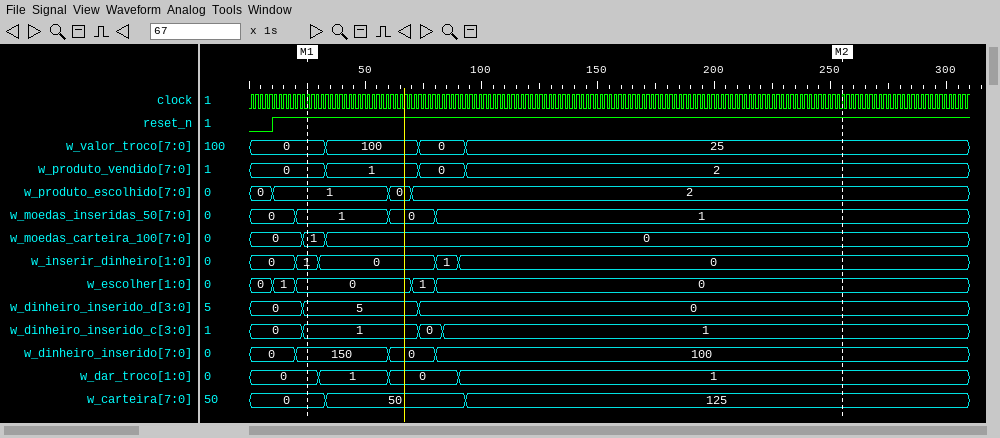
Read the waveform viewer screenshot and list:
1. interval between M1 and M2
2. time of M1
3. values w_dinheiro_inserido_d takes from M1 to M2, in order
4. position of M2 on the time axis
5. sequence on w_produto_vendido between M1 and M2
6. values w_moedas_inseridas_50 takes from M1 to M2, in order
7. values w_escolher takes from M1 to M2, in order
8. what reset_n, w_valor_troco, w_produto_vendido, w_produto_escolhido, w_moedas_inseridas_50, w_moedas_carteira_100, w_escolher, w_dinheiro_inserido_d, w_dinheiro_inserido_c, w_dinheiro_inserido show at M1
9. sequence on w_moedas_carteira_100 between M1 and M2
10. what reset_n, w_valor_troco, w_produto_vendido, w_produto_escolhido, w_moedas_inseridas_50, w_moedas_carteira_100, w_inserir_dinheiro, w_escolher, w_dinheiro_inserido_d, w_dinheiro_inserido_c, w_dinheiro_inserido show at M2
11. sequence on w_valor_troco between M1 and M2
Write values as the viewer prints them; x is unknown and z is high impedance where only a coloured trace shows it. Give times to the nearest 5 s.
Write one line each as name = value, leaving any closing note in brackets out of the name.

interval between M1 and M2 = 230 s
time of M1 = 25 s
values w_dinheiro_inserido_d takes from M1 to M2, in order = 5, 0
position of M2 on the time axis = 255 s
sequence on w_produto_vendido between M1 and M2 = 0, 1, 0, 2
values w_moedas_inseridas_50 takes from M1 to M2, in order = 1, 0, 1
values w_escolher takes from M1 to M2, in order = 0, 1, 0
what reset_n, w_valor_troco, w_produto_vendido, w_produto_escolhido, w_moedas_inseridas_50, w_moedas_carteira_100, w_escolher, w_dinheiro_inserido_d, w_dinheiro_inserido_c, w_dinheiro_inserido show at M1 = reset_n=1, w_valor_troco=0, w_produto_vendido=0, w_produto_escolhido=1, w_moedas_inseridas_50=1, w_moedas_carteira_100=1, w_escolher=0, w_dinheiro_inserido_d=5, w_dinheiro_inserido_c=1, w_dinheiro_inserido=150
sequence on w_moedas_carteira_100 between M1 and M2 = 1, 0
what reset_n, w_valor_troco, w_produto_vendido, w_produto_escolhido, w_moedas_inseridas_50, w_moedas_carteira_100, w_inserir_dinheiro, w_escolher, w_dinheiro_inserido_d, w_dinheiro_inserido_c, w_dinheiro_inserido show at M2 = reset_n=1, w_valor_troco=25, w_produto_vendido=2, w_produto_escolhido=2, w_moedas_inseridas_50=1, w_moedas_carteira_100=0, w_inserir_dinheiro=0, w_escolher=0, w_dinheiro_inserido_d=0, w_dinheiro_inserido_c=1, w_dinheiro_inserido=100
sequence on w_valor_troco between M1 and M2 = 0, 100, 0, 25
